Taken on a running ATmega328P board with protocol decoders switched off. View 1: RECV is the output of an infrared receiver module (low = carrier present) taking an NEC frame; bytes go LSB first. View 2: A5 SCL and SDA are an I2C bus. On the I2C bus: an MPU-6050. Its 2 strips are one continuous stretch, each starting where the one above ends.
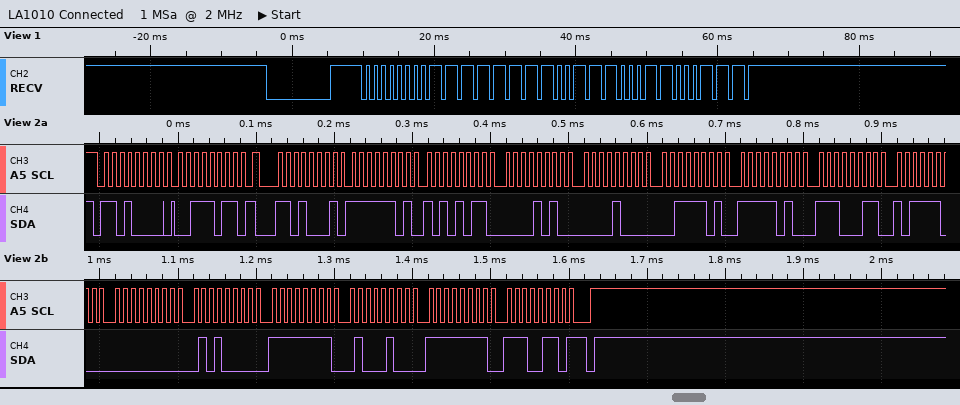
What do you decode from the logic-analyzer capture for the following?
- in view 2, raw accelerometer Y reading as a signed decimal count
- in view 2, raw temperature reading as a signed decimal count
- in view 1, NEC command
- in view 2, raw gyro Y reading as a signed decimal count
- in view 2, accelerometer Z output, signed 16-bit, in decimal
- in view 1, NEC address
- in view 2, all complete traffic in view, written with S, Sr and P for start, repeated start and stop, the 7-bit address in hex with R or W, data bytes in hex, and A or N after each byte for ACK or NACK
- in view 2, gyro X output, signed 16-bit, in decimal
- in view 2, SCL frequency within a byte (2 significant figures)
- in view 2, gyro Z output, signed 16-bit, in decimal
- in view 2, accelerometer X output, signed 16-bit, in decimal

2568
-7236
0x1C
-188
15866
0x00
S 68W A 3B A Sr 68R A FD A AB A 0A A 08 A 3D A FA A E3 A BC A 00 A 50 A FF A 44 A FF A E6 N P
80
100 kHz
-26
-597
